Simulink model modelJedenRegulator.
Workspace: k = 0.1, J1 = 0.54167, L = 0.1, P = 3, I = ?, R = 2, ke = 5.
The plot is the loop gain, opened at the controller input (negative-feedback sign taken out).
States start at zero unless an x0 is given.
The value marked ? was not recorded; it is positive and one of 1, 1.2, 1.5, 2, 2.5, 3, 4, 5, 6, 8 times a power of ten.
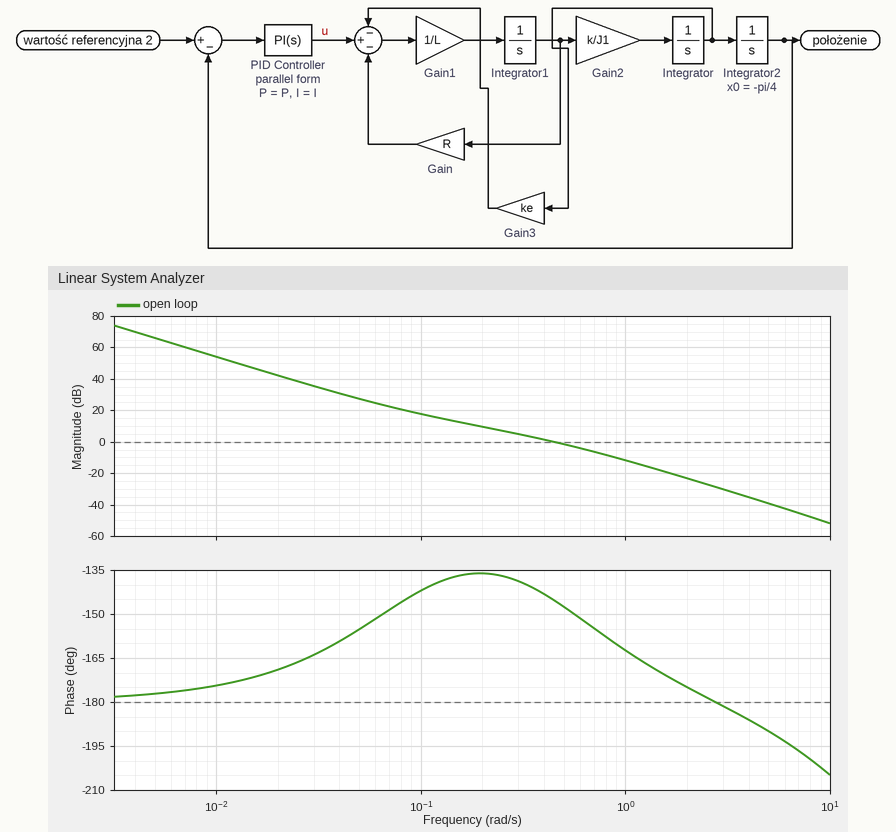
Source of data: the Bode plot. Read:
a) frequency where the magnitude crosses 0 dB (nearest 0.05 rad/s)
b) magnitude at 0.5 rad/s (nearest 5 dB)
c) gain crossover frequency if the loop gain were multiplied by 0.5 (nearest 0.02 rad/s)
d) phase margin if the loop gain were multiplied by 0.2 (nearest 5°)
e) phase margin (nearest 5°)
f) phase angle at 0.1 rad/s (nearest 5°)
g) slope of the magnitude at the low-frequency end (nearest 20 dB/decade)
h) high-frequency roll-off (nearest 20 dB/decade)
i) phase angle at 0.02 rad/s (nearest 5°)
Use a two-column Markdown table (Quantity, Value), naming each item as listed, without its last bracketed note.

| Quantity | Value |
|---|---|
| frequency where the magnitude crosses 0 dB | 0.45 rad/s |
| magnitude at 0.5 rad/s | 0 dB |
| gain crossover frequency if the loop gain were multiplied by 0.5 | 0.28 rad/s |
| phase margin if the loop gain were multiplied by 0.2 | 40° |
| phase margin | 35° |
| phase angle at 0.1 rad/s | -140° |
| slope of the magnitude at the low-frequency end | -40 dB/decade |
| high-frequency roll-off | -40 dB/decade |
| phase angle at 0.02 rad/s | -170° |
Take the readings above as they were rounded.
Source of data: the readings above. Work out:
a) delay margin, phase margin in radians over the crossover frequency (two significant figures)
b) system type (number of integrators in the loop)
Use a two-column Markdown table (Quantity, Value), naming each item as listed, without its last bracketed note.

| Quantity | Value |
|---|---|
| delay margin, phase margin in radians over the crossover frequency | 1.4 s |
| system type | 2 |
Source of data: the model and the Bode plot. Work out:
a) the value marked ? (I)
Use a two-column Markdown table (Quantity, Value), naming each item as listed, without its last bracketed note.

| Quantity | Value |
|---|---|
| the value marked ? | 0.25 |
